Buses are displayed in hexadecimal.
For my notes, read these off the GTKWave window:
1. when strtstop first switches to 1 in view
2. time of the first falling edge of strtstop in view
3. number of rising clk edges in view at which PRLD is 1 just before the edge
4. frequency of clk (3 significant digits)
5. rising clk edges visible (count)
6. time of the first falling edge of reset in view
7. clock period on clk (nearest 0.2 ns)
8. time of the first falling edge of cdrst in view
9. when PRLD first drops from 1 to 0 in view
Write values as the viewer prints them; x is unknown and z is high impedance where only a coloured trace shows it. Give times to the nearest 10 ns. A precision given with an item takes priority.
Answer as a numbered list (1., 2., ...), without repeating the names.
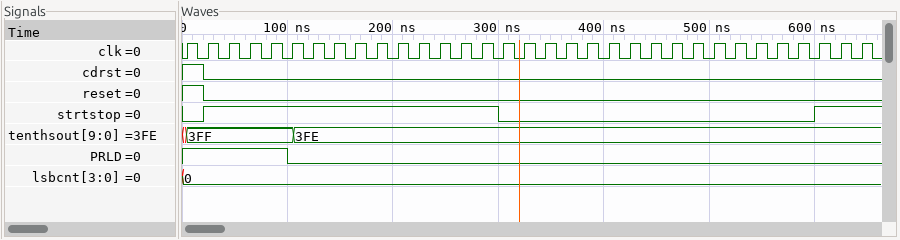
1. 20 ns
2. 300 ns
3. 5
4. 50.0 MHz
5. 33
6. 20 ns
7. 20 ns
8. 20 ns
9. 100 ns
